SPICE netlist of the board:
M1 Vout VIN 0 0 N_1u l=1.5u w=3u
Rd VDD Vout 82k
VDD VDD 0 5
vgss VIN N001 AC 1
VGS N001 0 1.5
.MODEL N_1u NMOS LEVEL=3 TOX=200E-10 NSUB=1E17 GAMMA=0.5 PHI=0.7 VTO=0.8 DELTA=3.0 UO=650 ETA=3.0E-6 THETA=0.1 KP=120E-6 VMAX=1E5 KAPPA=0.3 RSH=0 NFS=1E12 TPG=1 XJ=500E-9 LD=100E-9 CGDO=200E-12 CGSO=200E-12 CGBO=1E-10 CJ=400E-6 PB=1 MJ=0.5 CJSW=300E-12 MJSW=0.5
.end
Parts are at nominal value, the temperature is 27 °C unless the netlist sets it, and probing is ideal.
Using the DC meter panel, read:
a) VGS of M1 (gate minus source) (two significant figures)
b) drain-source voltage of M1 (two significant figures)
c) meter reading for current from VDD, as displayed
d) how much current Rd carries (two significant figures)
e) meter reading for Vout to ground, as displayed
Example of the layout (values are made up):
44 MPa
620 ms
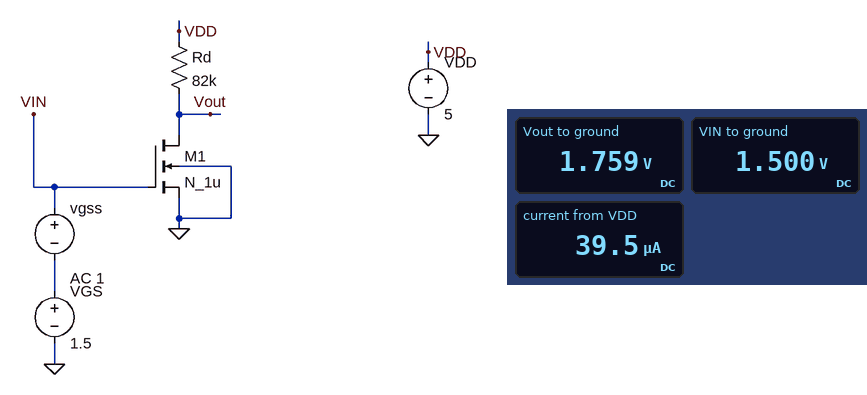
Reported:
1.5 V
1.8 V
39.5 µA
40 µA
1.759 V
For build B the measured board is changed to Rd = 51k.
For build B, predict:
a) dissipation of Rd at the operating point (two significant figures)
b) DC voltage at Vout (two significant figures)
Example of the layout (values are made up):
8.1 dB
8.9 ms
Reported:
83 µW
2.9 V
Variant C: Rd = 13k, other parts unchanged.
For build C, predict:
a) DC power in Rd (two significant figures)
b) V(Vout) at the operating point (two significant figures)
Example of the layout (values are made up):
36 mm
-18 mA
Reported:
22 µW
4.5 V
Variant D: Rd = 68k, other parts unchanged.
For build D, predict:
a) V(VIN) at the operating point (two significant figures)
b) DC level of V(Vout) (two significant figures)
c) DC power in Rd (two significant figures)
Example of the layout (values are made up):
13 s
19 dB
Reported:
1.5 V
2.3 V
110 µW
